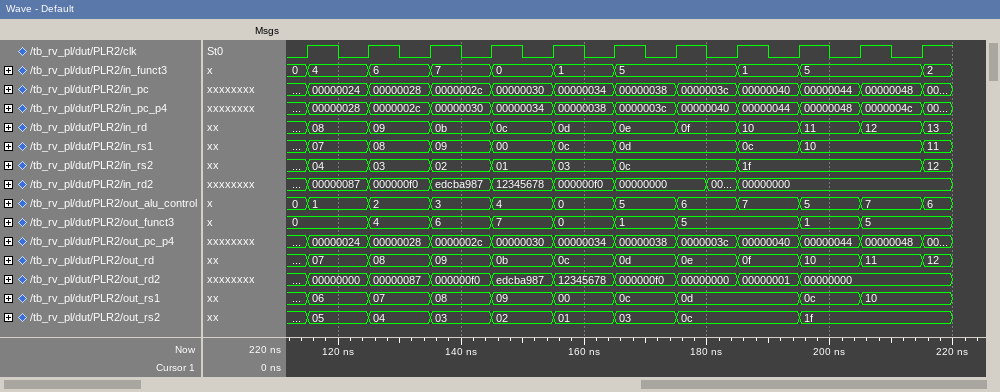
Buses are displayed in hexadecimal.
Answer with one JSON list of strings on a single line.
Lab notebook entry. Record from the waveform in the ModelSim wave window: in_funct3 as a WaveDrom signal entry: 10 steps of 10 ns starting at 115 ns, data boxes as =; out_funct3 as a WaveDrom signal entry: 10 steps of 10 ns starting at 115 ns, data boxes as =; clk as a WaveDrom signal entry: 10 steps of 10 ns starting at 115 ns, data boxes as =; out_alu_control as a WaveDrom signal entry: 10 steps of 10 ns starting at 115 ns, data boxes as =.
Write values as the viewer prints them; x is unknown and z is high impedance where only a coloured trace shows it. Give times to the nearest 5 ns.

["{name: 'in_funct3', wave: '======.==.', data: '4 6 7 0 1 5 1 5'}", "{name: 'out_funct3', wave: '=======.==', data: '0 4 6 7 0 1 5 1 5'}", "{name: 'clk', wave: 'p.........'}", "{name: 'out_alu_control', wave: '==========', data: '1 2 3 4 0 5 6 7 5 7'}"]
